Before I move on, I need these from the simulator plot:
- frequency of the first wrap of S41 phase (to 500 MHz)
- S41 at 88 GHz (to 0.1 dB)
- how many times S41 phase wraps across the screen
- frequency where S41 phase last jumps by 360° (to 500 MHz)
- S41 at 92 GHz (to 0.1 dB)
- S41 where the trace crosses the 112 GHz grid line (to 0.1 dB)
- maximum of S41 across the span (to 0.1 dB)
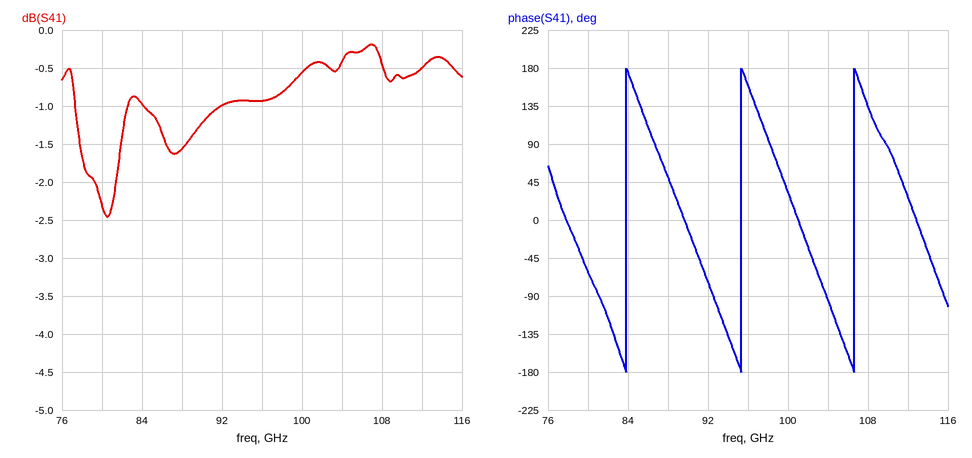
84.0 GHz
-1.6 dB
3
106.5 GHz
-1.0 dB
-0.5 dB
-0.2 dB
